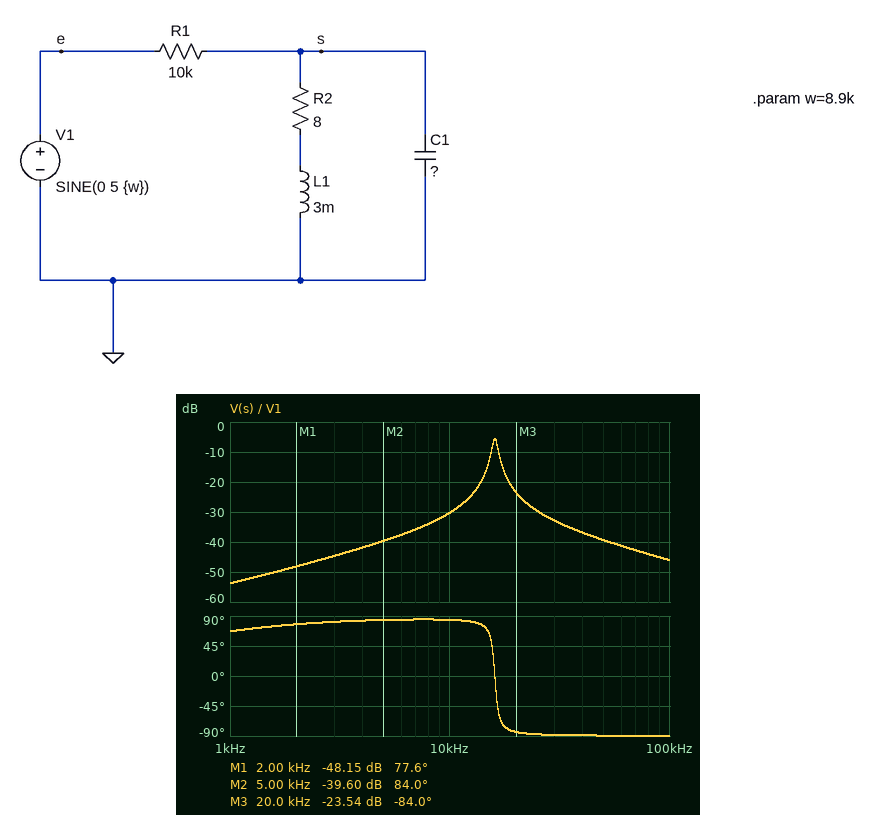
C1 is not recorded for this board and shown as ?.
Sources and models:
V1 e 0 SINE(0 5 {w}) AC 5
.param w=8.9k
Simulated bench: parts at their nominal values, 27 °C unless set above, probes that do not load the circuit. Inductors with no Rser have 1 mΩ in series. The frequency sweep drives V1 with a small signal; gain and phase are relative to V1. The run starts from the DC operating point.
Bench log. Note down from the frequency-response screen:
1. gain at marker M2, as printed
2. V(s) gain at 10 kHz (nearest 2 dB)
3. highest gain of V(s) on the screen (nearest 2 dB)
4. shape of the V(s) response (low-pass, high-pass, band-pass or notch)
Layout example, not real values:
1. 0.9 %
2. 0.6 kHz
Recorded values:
1. -39.60 dB
2. -30 dB
3. -6 dB
4. band-pass
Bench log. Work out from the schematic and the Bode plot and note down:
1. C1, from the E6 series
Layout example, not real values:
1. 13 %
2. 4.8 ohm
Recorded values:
1. 33 nF
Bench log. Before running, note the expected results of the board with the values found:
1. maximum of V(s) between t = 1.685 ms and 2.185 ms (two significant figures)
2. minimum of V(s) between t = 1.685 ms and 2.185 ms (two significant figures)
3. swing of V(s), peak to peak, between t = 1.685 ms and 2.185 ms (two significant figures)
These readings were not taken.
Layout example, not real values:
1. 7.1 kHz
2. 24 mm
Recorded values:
1. 120 mV
2. -120 mV
3. 240 mV
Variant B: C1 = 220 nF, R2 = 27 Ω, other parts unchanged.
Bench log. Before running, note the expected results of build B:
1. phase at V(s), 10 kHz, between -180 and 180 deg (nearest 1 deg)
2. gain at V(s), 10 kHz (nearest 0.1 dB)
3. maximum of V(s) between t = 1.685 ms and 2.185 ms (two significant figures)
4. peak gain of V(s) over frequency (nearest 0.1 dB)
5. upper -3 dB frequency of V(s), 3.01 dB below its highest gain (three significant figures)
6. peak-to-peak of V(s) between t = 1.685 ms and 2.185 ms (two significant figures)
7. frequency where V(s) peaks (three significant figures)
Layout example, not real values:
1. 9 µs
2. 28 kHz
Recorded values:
1. -84 deg
2. -38.8 dB
3. 76 mV
4. -26.1 dB
5. 6.99 kHz
6. 150 mV
7. 6.20 kHz
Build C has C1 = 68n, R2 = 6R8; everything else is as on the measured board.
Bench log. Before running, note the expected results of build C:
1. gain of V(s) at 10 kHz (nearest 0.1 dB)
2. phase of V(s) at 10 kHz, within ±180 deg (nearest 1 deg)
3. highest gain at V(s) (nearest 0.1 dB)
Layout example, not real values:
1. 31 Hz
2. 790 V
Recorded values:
1. -20.6 dB
2. 74 deg
3. -8.1 dB
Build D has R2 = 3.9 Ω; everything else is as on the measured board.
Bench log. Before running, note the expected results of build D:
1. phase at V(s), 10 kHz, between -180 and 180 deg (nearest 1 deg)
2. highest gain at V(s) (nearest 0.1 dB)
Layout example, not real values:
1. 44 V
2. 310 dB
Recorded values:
1. 86 deg
2. -3.1 dB
